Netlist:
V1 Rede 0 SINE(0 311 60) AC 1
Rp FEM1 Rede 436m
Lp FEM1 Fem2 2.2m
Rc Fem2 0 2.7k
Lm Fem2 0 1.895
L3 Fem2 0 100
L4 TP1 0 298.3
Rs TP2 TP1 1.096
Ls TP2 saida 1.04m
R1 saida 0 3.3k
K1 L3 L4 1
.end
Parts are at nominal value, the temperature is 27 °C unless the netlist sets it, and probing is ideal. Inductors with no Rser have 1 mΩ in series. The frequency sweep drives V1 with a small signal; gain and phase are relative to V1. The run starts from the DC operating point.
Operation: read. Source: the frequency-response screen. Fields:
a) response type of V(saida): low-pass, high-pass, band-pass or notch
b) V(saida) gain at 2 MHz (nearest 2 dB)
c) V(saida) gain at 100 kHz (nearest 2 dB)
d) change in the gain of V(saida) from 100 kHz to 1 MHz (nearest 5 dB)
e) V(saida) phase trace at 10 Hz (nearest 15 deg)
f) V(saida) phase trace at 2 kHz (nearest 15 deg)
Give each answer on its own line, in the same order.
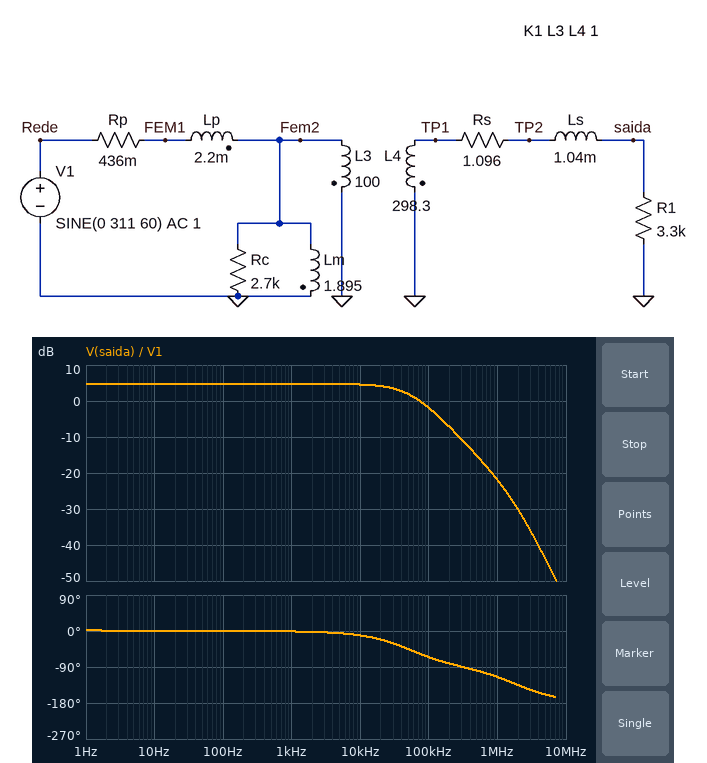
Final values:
low-pass
-30 dB
-2 dB
-20 dB
0 deg
0 deg
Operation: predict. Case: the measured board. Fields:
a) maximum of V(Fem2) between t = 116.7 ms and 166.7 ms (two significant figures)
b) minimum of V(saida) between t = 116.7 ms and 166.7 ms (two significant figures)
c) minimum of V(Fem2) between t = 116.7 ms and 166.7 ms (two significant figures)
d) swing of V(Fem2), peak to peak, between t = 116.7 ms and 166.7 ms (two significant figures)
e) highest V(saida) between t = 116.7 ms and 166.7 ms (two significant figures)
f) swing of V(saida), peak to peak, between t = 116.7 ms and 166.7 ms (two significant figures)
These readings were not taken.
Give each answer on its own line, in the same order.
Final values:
310 V
-540 V
-310 V
620 V
540 V
1.1 kV
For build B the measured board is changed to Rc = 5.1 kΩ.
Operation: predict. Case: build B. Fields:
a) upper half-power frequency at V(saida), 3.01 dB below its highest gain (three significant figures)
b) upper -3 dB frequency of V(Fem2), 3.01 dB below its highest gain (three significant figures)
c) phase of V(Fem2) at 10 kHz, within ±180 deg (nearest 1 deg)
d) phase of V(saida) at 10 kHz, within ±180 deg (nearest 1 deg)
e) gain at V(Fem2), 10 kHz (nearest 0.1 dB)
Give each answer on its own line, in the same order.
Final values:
59.4 kHz
60.2 kHz
-9 deg
-10 deg
-0.1 dB
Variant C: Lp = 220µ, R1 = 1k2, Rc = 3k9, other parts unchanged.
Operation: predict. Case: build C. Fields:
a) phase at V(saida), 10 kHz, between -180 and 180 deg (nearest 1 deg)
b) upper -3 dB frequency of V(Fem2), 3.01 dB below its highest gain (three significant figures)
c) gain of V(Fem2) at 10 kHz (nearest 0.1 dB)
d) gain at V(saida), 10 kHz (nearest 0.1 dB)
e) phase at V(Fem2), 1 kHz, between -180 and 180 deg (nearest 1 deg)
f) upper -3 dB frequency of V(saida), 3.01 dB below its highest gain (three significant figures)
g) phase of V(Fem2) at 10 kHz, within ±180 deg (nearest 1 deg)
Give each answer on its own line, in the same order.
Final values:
-5 deg
213 kHz
0 dB
4.7 dB
0 deg
111 kHz
-2 deg
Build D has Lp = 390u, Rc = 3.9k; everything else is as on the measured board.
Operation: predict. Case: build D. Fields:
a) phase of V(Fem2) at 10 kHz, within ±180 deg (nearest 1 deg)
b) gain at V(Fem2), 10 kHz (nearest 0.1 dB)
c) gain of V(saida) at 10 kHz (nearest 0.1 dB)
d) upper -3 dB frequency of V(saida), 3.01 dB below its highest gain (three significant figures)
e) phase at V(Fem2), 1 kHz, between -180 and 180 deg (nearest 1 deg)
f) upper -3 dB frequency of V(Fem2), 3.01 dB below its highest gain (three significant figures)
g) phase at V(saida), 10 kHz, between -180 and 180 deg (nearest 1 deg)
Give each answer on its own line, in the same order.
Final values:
-2 deg
0 dB
4.7 dB
219 kHz
0 deg
277 kHz
-3 deg
